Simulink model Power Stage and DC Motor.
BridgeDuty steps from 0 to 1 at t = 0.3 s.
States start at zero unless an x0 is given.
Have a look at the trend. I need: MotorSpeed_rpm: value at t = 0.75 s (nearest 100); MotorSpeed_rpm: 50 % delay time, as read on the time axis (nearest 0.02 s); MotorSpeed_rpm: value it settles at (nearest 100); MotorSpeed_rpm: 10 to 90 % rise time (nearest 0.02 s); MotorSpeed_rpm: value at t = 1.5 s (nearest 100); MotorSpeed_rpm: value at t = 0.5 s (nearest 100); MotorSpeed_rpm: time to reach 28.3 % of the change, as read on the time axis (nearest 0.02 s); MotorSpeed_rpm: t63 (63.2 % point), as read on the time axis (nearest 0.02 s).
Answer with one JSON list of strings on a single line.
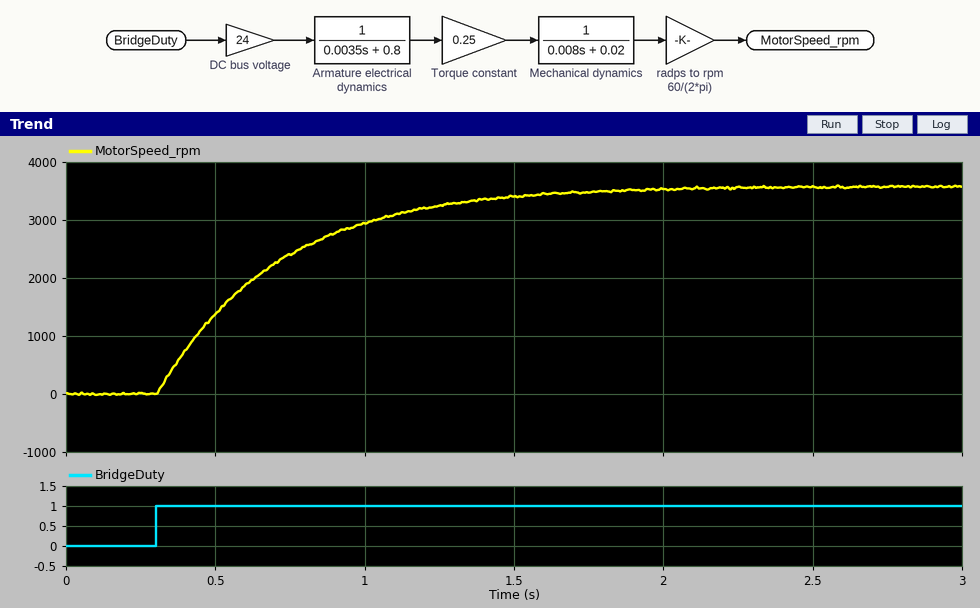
["2400", "0.58 s", "3600", "0.88 s", "3400", "1400", "0.44 s", "0.70 s"]
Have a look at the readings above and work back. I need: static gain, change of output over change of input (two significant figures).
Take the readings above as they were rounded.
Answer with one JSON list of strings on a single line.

["3600"]
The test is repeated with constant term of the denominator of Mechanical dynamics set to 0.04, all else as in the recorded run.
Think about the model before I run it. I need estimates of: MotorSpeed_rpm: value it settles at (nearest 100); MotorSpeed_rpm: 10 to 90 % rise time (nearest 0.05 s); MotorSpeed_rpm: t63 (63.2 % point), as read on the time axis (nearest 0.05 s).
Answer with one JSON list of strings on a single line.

["1800", "0.45 s", "0.50 s"]
